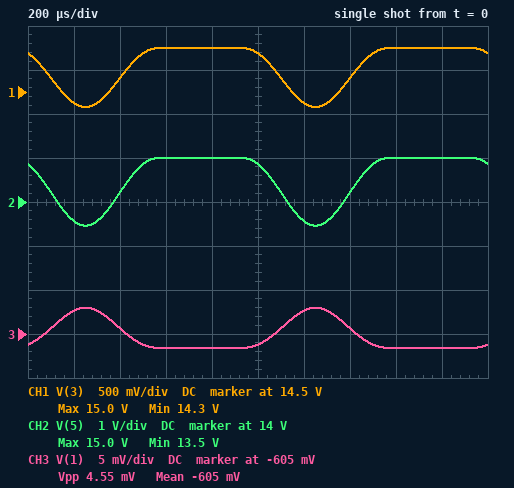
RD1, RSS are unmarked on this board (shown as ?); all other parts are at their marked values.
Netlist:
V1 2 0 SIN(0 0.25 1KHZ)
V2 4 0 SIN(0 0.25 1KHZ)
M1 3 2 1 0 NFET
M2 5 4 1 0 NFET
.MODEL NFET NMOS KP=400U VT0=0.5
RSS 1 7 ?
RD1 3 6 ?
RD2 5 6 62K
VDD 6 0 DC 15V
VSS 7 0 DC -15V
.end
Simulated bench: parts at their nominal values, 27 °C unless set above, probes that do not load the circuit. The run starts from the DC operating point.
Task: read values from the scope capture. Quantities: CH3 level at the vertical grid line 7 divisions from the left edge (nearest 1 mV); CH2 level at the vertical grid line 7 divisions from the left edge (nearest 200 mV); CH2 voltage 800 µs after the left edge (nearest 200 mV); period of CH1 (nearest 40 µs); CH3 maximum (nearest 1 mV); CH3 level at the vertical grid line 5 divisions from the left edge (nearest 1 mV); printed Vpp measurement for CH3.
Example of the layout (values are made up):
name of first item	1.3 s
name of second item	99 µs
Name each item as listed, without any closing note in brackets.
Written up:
CH3 level at the vertical grid line 7 divisions from the left edge	-604 mV
CH2 level at the vertical grid line 7 divisions from the left edge	14.2 V
CH2 voltage 800 µs after the left edge	15.0 V
period of CH1	1.00 ms
CH3 maximum	-602 mV
CH3 level at the vertical grid line 5 divisions from the left edge	-606 mV
printed Vpp measurement for CH3	4.55 mV
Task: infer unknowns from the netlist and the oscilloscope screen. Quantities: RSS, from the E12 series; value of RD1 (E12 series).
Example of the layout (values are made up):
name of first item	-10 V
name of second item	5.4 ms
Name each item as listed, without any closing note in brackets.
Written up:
RSS, from the E12 series	47 kΩ
value of RD1	27 kΩ
